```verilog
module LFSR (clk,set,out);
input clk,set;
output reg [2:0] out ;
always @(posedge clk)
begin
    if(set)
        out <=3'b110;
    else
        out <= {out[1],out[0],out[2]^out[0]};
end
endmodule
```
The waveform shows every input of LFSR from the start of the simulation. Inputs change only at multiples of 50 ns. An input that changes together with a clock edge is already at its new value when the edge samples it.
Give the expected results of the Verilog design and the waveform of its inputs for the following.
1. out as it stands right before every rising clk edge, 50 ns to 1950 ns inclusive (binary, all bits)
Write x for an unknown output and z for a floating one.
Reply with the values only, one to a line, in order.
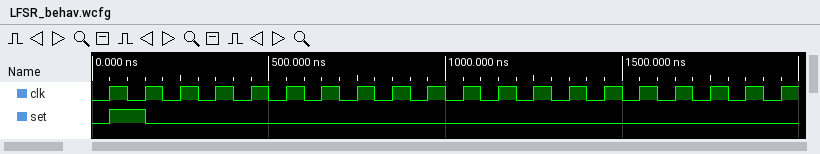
x, 110, 101, 010, 100, 001, 011, 111, 110, 101, 010, 100, 001, 011, 111, 110, 101, 010, 100, 001
